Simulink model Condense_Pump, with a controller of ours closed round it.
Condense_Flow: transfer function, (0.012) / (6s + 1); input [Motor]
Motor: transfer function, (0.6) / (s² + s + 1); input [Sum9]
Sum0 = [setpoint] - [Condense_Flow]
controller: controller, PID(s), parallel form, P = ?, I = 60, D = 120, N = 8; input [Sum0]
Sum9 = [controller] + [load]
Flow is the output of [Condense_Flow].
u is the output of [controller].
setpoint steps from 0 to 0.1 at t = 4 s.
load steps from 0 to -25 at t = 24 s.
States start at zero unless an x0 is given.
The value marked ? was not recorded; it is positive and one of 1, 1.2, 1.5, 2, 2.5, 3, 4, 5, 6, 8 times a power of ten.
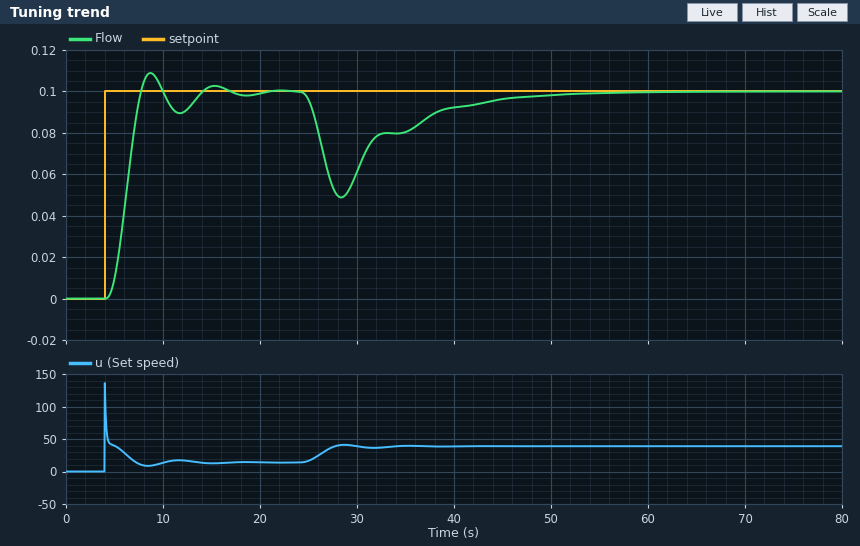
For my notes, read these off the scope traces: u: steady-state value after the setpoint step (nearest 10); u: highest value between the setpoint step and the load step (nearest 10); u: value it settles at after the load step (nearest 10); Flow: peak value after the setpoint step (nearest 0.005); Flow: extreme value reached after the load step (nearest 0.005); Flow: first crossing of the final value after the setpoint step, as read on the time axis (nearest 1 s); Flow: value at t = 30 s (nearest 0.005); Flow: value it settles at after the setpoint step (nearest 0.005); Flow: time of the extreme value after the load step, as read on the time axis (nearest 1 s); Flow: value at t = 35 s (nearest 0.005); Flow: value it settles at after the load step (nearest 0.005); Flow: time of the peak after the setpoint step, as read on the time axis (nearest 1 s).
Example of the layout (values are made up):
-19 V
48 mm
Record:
10
140
40
0.110
0.050
8 s
0.060
0.100
28 s
0.080
0.100
9 s
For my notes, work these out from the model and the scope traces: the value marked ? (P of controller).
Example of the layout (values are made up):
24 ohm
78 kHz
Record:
400
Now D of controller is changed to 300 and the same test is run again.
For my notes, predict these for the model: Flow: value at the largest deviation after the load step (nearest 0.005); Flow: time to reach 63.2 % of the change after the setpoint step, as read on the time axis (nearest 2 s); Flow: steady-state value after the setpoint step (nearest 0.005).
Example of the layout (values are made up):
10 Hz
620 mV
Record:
0.055
6 s
0.100
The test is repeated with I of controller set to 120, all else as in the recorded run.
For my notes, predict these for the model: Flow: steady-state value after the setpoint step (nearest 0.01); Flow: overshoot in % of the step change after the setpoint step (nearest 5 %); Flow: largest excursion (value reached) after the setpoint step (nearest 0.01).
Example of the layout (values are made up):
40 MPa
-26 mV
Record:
0.10
30 %
0.13
